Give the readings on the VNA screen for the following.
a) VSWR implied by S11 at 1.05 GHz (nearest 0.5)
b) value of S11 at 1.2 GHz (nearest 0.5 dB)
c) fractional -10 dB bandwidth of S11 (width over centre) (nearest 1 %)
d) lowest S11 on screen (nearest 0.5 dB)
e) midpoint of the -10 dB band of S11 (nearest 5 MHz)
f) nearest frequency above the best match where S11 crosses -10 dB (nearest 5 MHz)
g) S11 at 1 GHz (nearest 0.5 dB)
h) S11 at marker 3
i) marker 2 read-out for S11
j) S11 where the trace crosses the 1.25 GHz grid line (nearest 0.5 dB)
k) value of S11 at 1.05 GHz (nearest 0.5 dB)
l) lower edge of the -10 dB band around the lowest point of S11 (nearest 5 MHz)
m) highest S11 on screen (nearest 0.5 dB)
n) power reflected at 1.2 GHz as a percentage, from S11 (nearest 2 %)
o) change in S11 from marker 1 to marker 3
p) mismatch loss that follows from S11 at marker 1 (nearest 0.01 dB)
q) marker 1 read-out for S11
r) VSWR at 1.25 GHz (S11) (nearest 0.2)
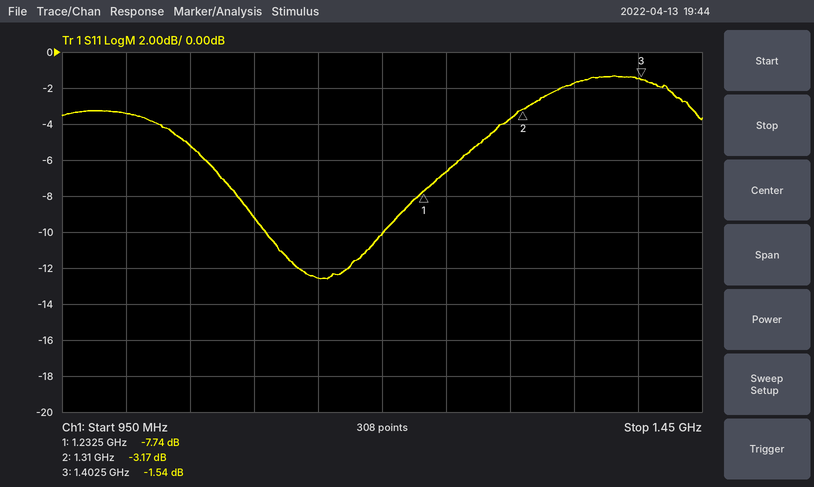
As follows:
3.5
-10.0 dB
8 %
-12.5 dB
1.155 GHz
1.200 GHz
-3.5 dB
-1.54 dB
-3.17 dB
-6.5 dB
-5.0 dB
1.110 GHz
-1.5 dB
10 %
6.20 dB
0.80 dB
-7.74 dB
2.8
